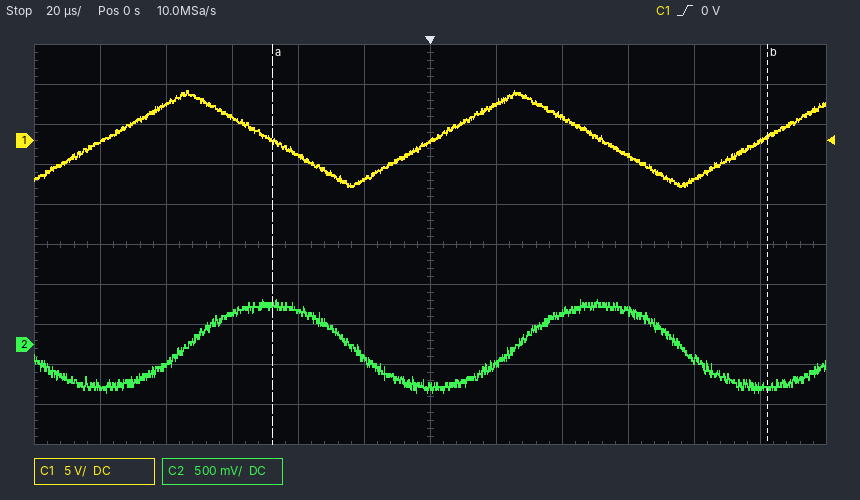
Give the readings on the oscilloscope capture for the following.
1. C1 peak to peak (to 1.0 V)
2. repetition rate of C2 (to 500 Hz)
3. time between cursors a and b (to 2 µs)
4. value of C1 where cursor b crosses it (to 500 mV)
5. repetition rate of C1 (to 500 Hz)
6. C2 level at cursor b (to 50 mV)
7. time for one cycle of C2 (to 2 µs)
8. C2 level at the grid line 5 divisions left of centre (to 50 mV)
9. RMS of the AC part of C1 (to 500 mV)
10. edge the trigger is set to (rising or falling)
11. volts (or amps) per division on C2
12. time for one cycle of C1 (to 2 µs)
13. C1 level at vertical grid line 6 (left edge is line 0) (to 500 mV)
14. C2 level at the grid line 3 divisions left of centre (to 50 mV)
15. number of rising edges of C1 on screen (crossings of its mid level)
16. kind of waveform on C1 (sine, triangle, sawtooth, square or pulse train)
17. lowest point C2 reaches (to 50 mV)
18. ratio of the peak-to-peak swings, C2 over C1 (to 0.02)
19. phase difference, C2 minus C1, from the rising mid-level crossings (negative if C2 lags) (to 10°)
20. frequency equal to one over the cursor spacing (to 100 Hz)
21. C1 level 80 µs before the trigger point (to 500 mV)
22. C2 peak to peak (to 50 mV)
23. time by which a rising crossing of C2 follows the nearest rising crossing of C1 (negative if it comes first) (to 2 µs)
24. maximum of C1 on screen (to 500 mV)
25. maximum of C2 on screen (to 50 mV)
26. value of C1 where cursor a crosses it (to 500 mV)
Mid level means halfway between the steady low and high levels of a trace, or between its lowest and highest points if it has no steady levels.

12.0 V
10.0 kHz
150 µs
500 mV
10.0 kHz
-550 mV
100 µs
-500 mV
3.5 V
rising
500 mV
100 µs
0.0 V
400 mV
3
triangle
-600 mV
0.10
-90°
6.7 kHz
4.5 V
1.15 V
+24 µs
6.0 V
550 mV
0.0 V
